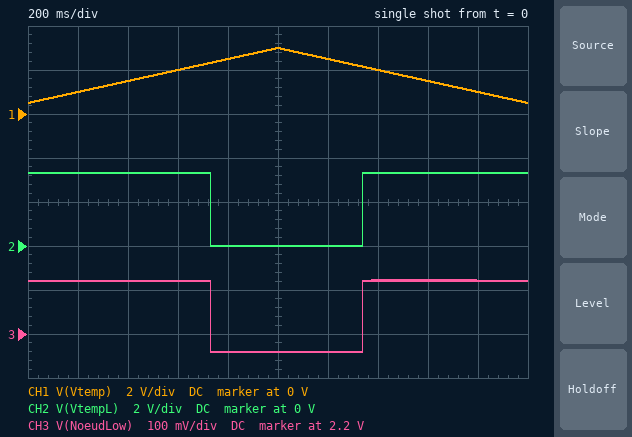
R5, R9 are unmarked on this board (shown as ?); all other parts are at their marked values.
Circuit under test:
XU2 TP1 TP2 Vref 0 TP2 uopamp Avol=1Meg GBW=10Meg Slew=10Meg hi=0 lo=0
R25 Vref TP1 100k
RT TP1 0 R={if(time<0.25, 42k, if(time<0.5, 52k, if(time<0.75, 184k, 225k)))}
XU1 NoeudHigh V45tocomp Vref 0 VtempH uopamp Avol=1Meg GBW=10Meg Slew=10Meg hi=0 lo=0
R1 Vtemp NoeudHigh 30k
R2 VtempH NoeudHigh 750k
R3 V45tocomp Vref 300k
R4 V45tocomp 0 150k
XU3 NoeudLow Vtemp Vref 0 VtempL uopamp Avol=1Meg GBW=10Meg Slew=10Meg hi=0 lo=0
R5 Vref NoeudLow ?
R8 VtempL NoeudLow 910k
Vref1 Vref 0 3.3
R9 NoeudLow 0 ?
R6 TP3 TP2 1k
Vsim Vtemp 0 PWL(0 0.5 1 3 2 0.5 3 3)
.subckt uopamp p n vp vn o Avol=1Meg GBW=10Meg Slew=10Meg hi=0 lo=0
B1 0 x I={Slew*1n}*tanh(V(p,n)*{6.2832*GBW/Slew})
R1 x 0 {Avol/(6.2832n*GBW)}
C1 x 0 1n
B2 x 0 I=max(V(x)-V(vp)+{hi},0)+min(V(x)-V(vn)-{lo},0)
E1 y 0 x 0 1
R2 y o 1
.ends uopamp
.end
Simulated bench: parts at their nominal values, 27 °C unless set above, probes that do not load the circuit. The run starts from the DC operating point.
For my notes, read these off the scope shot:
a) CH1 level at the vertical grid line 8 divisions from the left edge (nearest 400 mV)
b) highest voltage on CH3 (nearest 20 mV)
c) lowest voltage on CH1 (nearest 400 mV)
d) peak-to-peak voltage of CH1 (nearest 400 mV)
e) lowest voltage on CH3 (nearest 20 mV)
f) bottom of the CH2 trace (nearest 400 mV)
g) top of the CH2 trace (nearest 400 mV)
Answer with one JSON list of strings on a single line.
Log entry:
["1.6 V", "2.32 V", "400 mV", "2.4 V", "2.16 V", "0 V", "3.2 V"]
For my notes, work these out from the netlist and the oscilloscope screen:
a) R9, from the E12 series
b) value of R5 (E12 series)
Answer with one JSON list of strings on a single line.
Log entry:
["150 kΩ", "68 kΩ"]
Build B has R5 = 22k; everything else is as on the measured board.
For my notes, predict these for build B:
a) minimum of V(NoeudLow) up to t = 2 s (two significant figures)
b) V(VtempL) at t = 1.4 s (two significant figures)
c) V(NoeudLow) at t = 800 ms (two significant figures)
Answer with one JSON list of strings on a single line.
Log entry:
["2.8 V", "3.3 V", "2.9 V"]
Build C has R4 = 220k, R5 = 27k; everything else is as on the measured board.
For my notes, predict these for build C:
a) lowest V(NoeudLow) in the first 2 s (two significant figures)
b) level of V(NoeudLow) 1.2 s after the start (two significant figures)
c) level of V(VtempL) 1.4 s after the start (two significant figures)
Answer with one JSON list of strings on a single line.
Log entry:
["2.7 V", "2.8 V", "3.3 V"]
